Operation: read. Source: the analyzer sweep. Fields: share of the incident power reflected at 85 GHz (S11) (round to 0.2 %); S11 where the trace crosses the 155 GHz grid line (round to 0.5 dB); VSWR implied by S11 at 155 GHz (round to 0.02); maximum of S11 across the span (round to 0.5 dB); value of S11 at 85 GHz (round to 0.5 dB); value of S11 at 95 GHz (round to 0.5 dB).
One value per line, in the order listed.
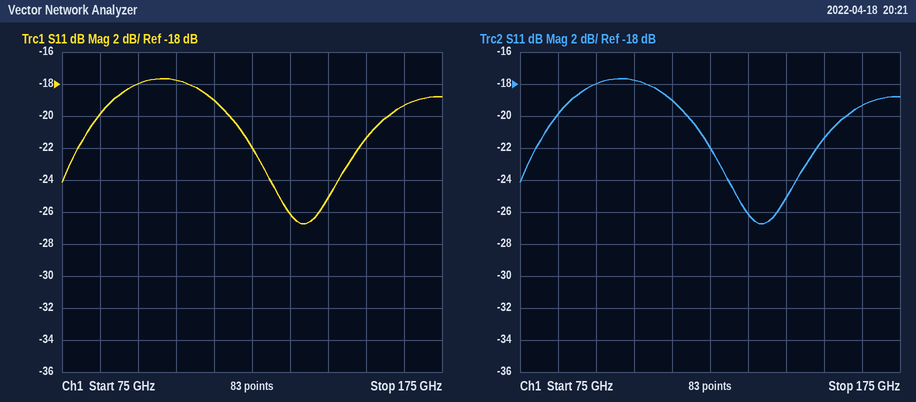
1.0 %
-21.5 dB
1.18
-17.5 dB
-20.0 dB
-18.0 dB
